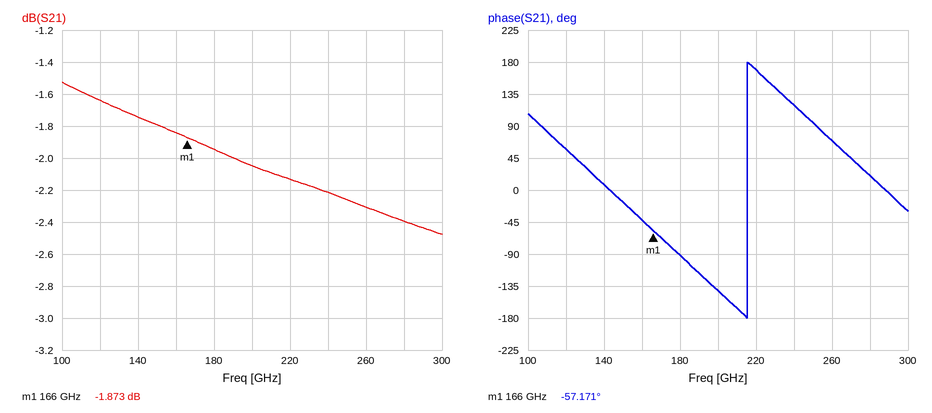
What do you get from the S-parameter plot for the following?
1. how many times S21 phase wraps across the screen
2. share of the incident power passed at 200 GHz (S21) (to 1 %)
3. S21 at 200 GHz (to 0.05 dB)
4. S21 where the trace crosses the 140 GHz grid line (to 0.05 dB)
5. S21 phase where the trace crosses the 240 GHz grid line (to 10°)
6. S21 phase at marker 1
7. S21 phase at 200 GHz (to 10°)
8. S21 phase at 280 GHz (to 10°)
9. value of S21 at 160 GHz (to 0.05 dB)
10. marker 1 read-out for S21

1
62 %
-2.05 dB
-1.75 dB
120°
-57.171°
-140°
20°
-1.85 dB
-1.873 dB
